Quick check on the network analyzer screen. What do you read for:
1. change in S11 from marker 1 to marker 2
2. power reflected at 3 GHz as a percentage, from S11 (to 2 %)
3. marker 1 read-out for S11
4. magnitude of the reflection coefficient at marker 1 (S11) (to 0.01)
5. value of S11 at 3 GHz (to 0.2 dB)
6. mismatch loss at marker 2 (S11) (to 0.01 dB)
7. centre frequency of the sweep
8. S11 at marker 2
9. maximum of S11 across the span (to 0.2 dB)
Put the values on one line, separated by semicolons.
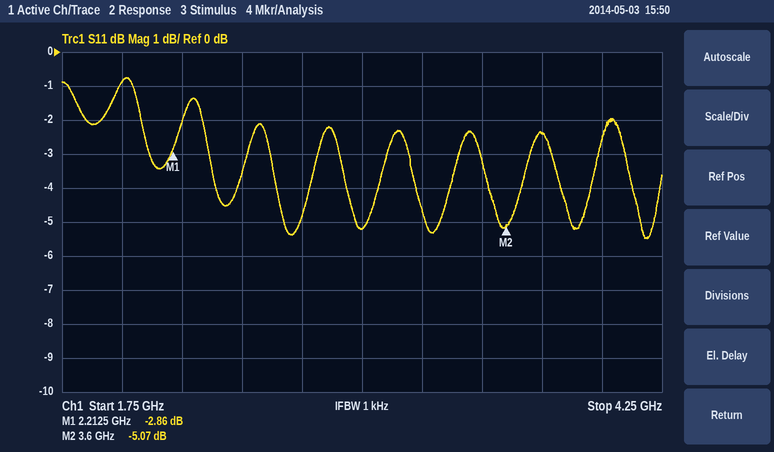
-2.21 dB; 30 %; -2.86 dB; 0.72; -5.2 dB; 1.62 dB; 3 GHz; -5.07 dB; -0.8 dB
